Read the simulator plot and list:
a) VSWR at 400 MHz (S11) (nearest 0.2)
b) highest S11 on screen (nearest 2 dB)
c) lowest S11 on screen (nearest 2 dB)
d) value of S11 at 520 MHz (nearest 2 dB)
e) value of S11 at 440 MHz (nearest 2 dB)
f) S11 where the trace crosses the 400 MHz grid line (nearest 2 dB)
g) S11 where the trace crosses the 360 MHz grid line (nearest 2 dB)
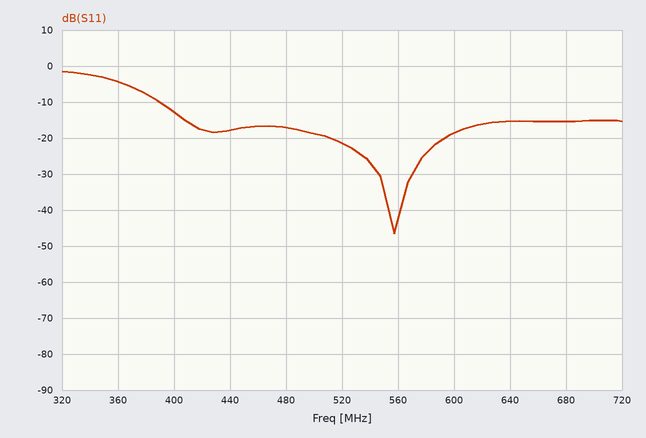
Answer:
1.6
-2 dB
-46 dB
-22 dB
-18 dB
-12 dB
-4 dB
